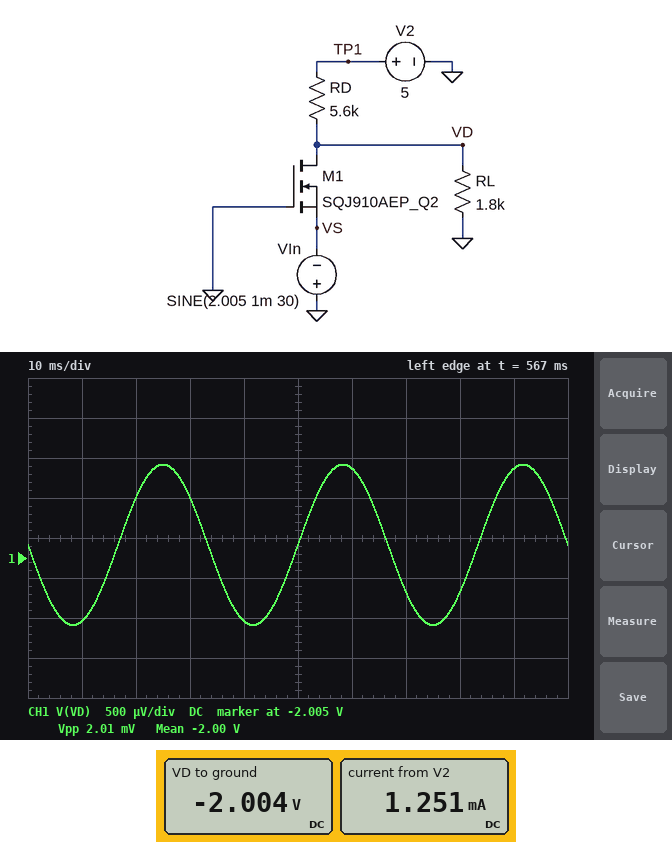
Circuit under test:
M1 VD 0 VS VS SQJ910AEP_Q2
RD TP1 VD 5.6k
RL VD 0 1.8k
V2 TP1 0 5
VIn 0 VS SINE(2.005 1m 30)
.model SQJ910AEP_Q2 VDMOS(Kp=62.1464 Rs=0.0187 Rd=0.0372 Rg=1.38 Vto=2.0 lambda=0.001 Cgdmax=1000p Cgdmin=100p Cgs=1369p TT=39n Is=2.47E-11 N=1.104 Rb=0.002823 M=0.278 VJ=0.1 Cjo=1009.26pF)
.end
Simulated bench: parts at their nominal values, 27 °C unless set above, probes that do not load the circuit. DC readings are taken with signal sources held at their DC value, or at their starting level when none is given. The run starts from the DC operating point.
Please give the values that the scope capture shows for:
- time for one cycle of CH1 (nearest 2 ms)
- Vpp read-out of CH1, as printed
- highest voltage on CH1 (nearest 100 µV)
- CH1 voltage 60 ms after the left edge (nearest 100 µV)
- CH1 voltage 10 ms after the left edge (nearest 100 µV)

34 ms
2.01 mV
-2.0033 V
-2.0034 V
-2.0053 V
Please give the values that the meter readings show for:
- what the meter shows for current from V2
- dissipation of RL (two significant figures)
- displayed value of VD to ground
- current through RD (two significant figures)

1.251 mA
2.2 mW
-2.004 V
1.3 mA
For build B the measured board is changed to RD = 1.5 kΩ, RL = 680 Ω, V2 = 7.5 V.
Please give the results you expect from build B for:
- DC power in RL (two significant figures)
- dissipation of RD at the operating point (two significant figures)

5.9 mW
60 mW
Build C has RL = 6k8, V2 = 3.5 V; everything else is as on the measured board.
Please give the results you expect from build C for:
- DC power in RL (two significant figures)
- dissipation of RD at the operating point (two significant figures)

590 µW
5.4 mW
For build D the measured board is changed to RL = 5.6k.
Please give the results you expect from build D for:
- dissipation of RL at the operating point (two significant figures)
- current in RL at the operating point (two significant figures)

720 µW
360 µA
